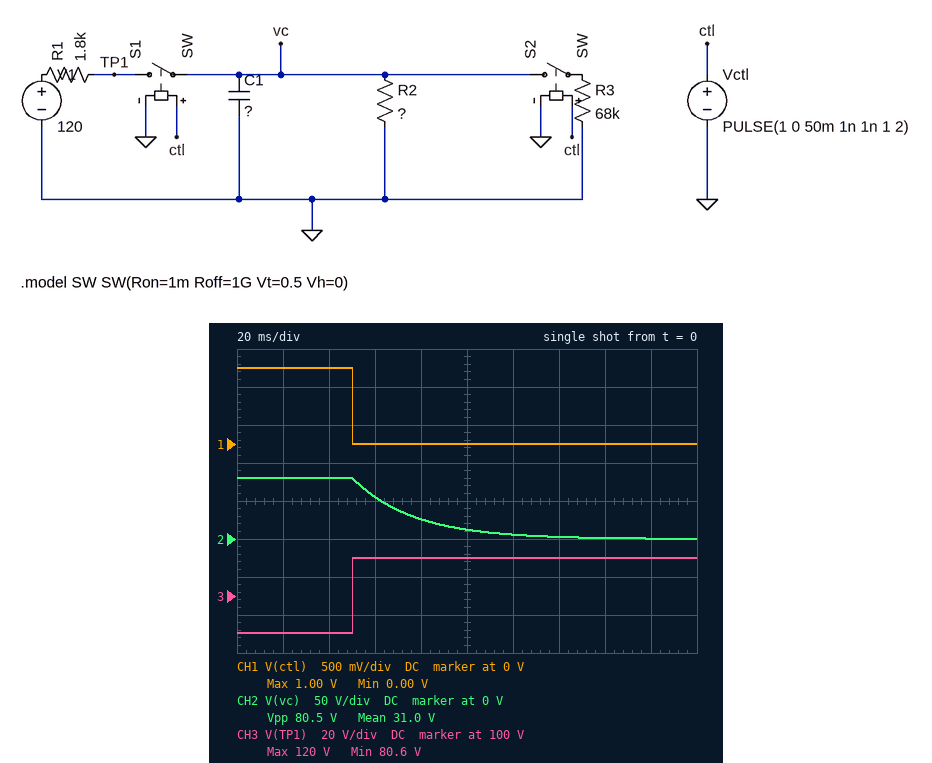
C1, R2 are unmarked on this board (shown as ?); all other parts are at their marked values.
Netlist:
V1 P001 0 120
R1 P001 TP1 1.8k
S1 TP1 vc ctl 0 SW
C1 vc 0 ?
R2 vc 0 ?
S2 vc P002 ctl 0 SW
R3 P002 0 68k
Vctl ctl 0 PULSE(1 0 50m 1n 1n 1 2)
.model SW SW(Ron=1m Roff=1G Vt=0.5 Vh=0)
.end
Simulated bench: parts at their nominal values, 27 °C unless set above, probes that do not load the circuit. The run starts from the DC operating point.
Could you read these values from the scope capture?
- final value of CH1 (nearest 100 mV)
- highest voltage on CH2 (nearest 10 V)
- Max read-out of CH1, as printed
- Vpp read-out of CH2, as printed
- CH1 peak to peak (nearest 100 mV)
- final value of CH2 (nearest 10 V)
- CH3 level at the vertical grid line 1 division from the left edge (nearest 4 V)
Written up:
0 V
80 V
1.00 V
80.5 V
1.0 V
0 V
80 V
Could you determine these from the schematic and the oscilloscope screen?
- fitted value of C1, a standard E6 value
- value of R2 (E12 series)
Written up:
6.8 µF
3.9 kΩ
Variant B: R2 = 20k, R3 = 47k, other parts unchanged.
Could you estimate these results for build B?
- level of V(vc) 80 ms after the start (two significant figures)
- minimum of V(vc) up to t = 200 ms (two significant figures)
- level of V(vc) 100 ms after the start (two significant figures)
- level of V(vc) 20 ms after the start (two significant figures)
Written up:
85 V
35 V
74 V
110 V
